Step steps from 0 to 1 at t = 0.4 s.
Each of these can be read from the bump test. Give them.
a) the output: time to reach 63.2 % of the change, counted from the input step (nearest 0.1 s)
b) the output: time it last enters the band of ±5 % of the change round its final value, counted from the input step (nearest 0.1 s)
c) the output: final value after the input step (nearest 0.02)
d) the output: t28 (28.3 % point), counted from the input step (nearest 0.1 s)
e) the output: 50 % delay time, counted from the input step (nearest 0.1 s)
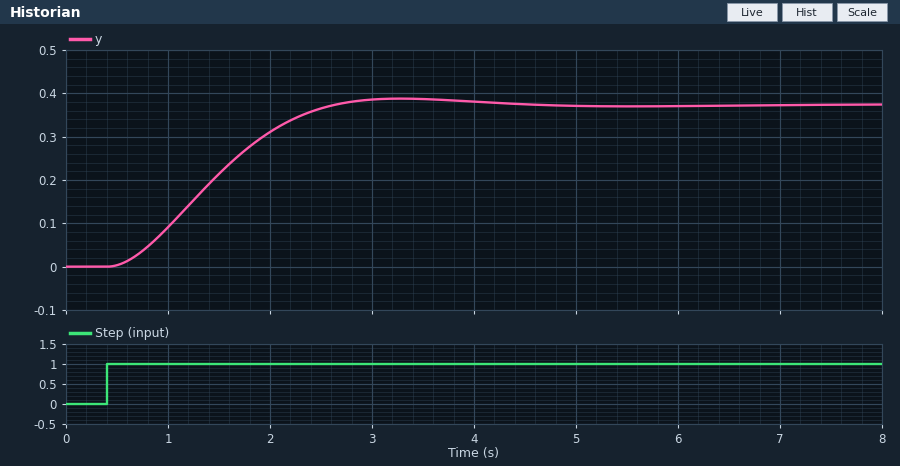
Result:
1.2 s
2.0 s
0.38
0.7 s
1.0 s
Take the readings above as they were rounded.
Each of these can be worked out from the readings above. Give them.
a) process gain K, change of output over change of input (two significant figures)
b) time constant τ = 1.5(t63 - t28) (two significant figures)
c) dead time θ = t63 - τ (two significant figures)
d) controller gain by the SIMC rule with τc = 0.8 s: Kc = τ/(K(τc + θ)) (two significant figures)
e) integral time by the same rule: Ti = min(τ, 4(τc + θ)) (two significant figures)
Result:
0.38
0.75 s
0.45 s
1.6
0.75 s
